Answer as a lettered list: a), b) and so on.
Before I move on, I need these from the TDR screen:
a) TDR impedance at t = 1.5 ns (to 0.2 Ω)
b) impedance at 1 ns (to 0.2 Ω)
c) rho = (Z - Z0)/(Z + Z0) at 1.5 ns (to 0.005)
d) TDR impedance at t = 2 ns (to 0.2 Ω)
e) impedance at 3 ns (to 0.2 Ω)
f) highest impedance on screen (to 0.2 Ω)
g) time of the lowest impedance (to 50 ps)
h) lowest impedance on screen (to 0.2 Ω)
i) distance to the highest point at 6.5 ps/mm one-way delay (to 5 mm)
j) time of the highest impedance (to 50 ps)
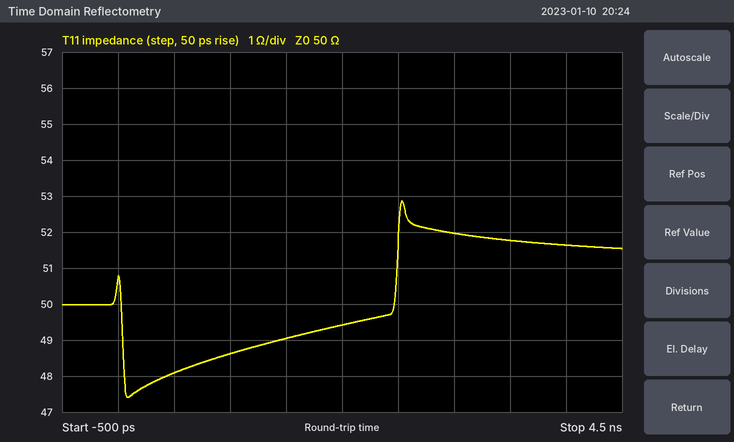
a) 49.0 Ω
b) 48.6 Ω
c) -0.010
d) 49.4 Ω
e) 52.0 Ω
f) 52.8 Ω
g) 100 ps
h) 47.4 Ω
i) 195 mm
j) 2.55 ns
